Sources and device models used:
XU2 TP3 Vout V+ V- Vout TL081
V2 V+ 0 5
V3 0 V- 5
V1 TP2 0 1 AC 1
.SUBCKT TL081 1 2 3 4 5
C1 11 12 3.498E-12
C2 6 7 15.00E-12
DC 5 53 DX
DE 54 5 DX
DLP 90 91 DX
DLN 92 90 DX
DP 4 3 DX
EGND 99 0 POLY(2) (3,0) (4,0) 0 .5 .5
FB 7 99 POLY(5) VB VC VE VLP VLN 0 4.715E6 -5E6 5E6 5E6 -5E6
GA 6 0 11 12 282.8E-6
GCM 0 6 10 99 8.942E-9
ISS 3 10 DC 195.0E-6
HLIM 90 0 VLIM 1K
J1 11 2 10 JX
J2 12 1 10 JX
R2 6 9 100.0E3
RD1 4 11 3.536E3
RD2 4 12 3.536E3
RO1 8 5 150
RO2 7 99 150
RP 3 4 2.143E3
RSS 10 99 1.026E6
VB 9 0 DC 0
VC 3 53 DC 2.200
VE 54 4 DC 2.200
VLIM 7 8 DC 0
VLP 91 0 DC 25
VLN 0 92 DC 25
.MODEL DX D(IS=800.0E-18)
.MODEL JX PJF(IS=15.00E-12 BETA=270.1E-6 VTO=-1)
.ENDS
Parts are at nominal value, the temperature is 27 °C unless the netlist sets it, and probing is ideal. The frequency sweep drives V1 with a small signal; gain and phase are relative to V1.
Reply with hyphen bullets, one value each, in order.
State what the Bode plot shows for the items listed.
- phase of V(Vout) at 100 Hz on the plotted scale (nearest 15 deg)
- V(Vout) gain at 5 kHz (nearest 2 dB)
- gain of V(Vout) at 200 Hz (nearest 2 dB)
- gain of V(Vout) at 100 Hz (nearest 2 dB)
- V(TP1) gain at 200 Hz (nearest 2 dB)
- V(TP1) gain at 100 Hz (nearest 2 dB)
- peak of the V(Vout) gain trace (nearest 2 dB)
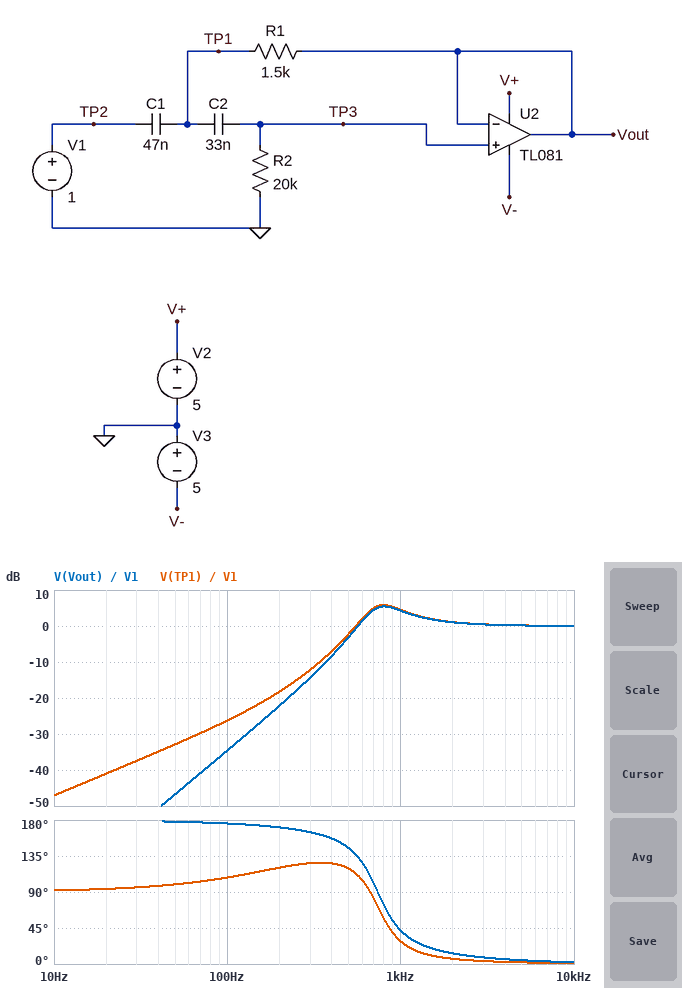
- 180 deg
- 0 dB
- -22 dB
- -34 dB
- -18 dB
- -26 dB
- 6 dB
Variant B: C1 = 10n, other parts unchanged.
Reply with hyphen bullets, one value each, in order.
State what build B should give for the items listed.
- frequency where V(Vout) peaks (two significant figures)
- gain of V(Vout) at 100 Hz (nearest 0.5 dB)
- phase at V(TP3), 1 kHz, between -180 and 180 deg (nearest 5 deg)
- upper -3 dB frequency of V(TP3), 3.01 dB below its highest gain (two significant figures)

- 1.8 kHz
- -48.0 dB
- 145 deg
- 3.8 kHz
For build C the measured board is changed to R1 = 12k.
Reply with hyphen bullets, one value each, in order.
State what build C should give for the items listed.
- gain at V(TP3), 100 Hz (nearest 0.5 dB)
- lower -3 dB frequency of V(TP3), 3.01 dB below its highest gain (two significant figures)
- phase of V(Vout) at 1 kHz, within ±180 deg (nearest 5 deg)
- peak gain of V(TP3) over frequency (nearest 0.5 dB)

- -17.0 dB
- 290 Hz
- 25 deg
- 0 dB
